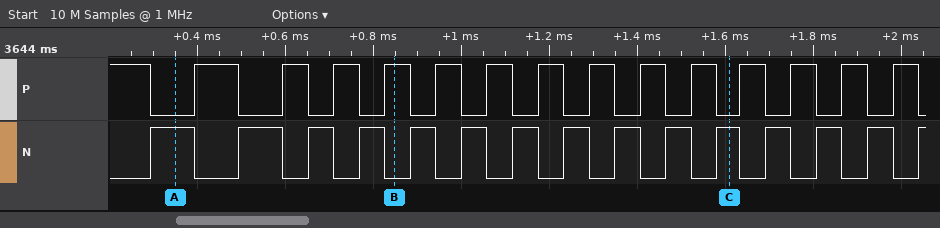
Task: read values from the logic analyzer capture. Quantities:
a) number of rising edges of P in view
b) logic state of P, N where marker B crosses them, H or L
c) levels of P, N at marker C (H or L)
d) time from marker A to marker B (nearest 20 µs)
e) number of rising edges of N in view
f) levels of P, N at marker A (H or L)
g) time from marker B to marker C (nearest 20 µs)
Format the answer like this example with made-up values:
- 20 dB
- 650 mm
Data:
- 14
- P=H, N=L
- P=L, N=H
- 500 µs
- 15
- P=L, N=H
- 760 µs
